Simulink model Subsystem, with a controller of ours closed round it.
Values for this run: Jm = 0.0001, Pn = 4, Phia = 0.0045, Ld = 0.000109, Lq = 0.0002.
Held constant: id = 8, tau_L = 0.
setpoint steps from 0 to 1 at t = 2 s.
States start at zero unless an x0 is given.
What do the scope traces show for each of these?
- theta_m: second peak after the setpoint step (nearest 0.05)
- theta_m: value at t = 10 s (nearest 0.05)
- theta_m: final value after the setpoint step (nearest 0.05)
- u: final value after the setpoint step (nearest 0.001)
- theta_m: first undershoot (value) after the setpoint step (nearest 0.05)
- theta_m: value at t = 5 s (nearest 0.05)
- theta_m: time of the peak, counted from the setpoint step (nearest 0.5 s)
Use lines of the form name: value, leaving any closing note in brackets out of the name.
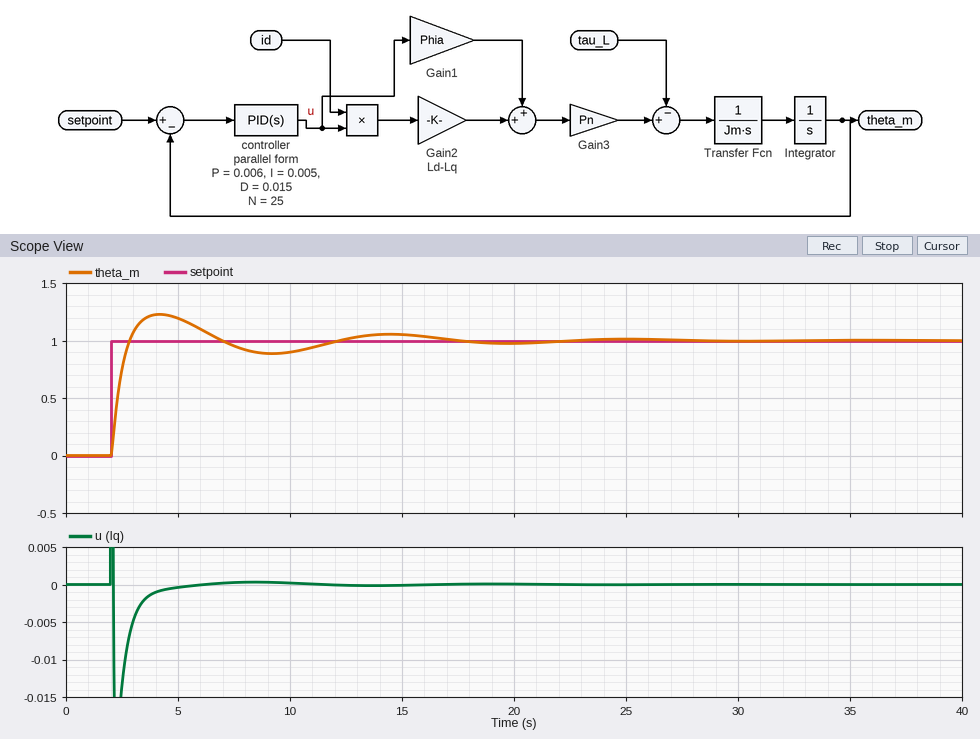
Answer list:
theta_m: second peak after the setpoint step: 1.05
theta_m: value at t = 10 s: 0.90
theta_m: final value after the setpoint step: 1.00
u: final value after the setpoint step: 0.000
theta_m: first undershoot (value) after the setpoint step: 0.90
theta_m: value at t = 5 s: 1.20
theta_m: time of the peak, counted from the setpoint step: 2.0 s
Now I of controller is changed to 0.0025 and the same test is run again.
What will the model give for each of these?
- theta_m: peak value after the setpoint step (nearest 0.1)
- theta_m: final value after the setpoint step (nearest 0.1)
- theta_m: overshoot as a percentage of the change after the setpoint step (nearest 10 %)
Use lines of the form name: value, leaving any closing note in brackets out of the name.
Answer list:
theta_m: peak value after the setpoint step: 1.2
theta_m: final value after the setpoint step: 1.0
theta_m: overshoot as a percentage of the change after the setpoint step: 20 %
